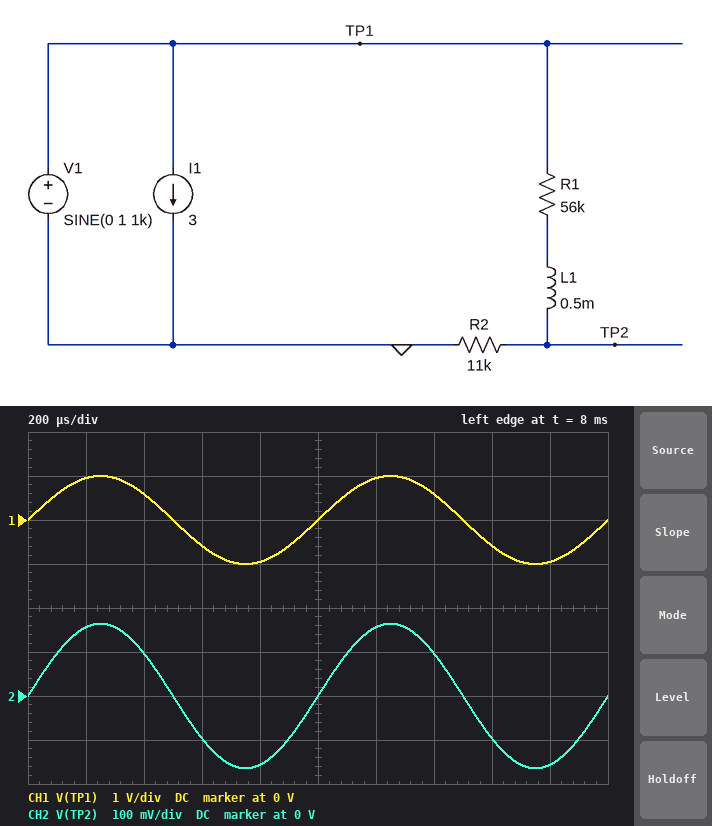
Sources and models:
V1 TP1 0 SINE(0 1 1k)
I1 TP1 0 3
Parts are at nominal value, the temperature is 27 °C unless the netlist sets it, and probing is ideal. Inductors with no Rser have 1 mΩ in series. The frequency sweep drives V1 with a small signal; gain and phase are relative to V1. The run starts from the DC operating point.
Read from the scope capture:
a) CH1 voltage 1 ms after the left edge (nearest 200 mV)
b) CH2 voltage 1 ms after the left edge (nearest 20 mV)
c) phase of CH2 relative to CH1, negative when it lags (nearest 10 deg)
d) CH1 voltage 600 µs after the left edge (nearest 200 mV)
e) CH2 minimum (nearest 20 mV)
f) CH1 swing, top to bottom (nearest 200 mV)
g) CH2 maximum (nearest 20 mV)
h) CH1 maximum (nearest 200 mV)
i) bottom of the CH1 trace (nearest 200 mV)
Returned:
0 V
0 V
0 deg
-600 mV
-160 mV
2.0 V
160 mV
1.0 V
-1.0 V
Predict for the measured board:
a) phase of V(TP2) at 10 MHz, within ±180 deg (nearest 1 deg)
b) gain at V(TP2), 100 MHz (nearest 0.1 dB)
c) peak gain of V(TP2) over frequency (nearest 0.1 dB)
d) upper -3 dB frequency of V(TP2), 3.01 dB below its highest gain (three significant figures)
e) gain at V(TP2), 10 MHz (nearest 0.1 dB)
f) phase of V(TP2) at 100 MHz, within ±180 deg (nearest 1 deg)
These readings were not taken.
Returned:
-25 deg
-29.3 dB
-15.7 dB
21.3 MHz
-16.6 dB
-78 deg
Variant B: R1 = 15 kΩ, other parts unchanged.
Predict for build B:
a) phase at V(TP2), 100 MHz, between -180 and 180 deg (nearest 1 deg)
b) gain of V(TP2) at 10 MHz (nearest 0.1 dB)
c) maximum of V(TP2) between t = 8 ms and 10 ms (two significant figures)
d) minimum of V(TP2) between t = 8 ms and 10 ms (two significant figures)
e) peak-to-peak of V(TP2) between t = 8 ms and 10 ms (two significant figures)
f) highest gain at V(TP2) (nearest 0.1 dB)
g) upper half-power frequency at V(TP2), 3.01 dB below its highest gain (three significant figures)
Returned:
-85 deg
-11.4 dB
420 mV
-420 mV
850 mV
-7.5 dB
8.28 MHz
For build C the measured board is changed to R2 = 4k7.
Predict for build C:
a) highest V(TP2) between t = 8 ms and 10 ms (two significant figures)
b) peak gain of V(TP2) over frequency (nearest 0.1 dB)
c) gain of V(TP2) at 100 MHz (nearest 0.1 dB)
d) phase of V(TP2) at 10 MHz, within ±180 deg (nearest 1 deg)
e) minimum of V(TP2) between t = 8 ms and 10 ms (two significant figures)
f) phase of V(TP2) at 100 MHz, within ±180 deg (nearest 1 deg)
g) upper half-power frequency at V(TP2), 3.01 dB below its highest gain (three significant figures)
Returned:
77 mV
-22.2 dB
-36.7 dB
-27 deg
-77 mV
-79 deg
19.3 MHz
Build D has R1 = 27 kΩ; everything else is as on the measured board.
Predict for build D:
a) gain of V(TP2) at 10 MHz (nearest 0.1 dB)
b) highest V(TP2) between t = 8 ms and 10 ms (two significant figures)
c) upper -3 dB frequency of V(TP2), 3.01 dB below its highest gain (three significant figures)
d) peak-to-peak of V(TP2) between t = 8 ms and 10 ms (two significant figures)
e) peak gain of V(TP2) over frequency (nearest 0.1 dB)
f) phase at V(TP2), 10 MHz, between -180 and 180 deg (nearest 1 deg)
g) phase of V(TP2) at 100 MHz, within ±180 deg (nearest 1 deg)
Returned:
-13.0 dB
290 mV
12.1 MHz
580 mV
-10.8 dB
-40 deg
-83 deg
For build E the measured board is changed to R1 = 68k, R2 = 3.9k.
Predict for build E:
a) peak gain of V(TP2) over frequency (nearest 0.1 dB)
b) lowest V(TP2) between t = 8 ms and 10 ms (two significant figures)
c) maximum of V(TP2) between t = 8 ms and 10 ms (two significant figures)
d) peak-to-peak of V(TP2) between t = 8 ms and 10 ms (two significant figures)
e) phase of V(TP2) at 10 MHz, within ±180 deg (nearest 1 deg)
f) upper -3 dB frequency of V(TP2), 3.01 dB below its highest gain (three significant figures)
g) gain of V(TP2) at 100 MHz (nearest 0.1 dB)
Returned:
-25.3 dB
-54 mV
54 mV
110 mV
-24 deg
22.9 MHz
-38.3 dB
